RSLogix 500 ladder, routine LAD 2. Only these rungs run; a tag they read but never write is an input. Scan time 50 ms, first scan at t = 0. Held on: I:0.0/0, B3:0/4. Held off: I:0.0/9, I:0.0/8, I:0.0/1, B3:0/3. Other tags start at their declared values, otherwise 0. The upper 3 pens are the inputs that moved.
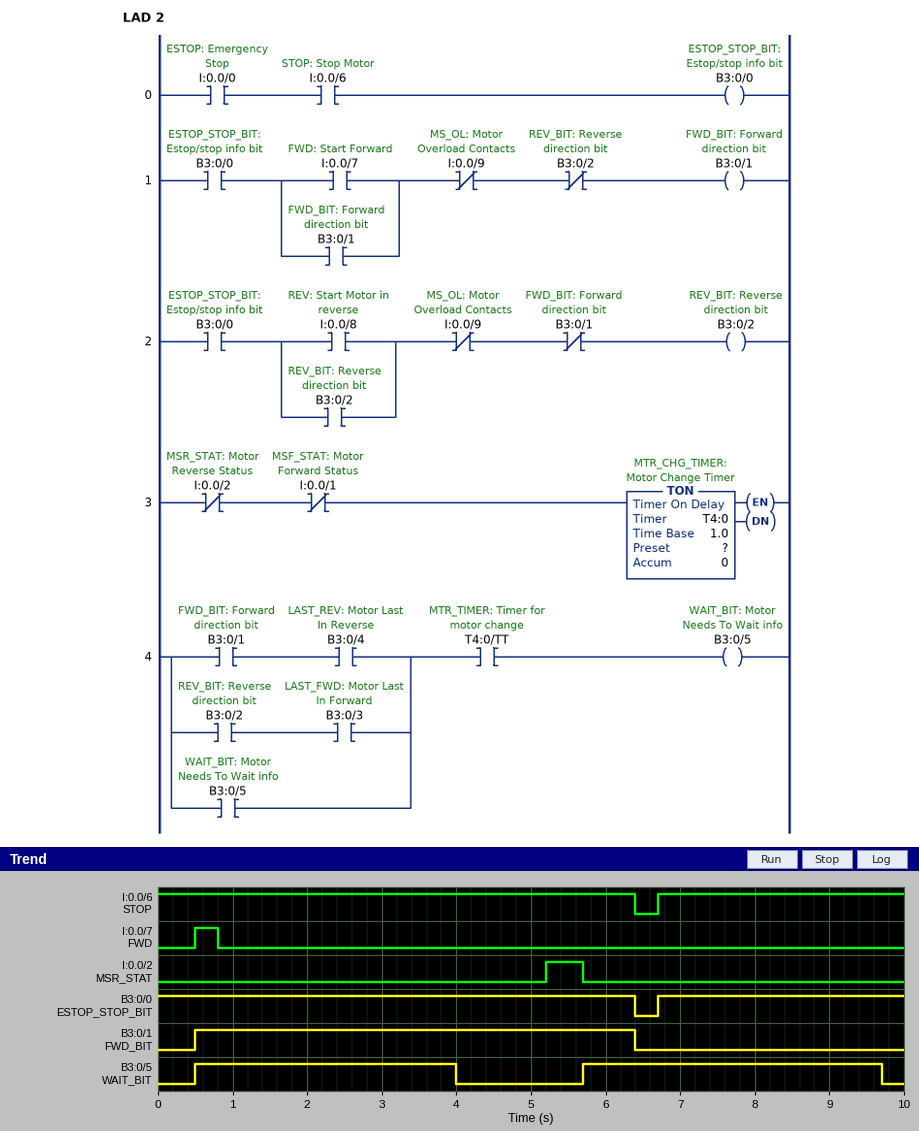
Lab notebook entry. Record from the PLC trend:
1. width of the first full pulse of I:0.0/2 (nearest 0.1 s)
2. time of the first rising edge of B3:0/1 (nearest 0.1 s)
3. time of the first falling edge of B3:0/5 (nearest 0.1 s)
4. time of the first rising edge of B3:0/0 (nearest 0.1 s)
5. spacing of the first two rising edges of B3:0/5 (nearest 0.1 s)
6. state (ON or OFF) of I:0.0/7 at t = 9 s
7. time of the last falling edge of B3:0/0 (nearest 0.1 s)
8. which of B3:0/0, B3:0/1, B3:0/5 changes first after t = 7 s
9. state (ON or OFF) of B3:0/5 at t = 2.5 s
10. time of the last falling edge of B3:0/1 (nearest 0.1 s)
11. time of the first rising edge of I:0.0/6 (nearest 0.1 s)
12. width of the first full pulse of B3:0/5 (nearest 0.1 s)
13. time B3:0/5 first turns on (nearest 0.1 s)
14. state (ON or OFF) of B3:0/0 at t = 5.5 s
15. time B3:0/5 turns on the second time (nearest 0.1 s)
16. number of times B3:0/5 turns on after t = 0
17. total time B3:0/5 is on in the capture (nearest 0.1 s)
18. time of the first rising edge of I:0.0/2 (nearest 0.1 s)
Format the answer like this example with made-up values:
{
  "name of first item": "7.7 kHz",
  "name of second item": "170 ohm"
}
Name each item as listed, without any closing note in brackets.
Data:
{
  "width of the first full pulse of I:0.0/2": "0.5 s",
  "time of the first rising edge of B3:0/1": "0.5 s",
  "time of the first falling edge of B3:0/5": "4.0 s",
  "time of the first rising edge of B3:0/0": "6.7 s",
  "spacing of the first two rising edges of B3:0/5": "5.2 s",
  "state (ON or OFF) of I:0.0/7 at t = 9 s": "OFF",
  "time of the last falling edge of B3:0/0": "6.4 s",
  "which of B3:0/0, B3:0/1, B3:0/5 changes first after t = 7 s": "B3:0/5",
  "state (ON or OFF) of B3:0/5 at t = 2.5 s": "ON",
  "time of the last falling edge of B3:0/1": "6.4 s",
  "time of the first rising edge of I:0.0/6": "6.7 s",
  "width of the first full pulse of B3:0/5": "3.5 s",
  "time B3:0/5 first turns on": "0.5 s",
  "state (ON or OFF) of B3:0/0 at t = 5.5 s": "ON",
  "time B3:0/5 turns on the second time": "5.7 s",
  "number of times B3:0/5 turns on after t = 0": "2",
  "total time B3:0/5 is on in the capture": "7.5 s",
  "time of the first rising edge of I:0.0/2": "5.2 s"
}
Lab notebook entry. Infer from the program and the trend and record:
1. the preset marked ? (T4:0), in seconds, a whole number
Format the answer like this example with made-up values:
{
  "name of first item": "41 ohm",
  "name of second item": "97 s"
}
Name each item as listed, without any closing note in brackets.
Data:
{
  "the preset marked ? (T4:0), in seconds, a whole number": "4 s"
}
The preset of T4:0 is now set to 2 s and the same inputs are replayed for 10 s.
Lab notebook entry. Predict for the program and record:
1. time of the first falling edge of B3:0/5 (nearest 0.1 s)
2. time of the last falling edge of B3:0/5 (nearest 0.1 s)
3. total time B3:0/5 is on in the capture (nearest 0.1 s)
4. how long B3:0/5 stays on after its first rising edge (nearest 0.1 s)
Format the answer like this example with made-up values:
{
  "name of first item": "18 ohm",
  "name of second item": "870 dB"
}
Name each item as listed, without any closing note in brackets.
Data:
{
  "time of the first falling edge of B3:0/5": "2.0 s",
  "time of the last falling edge of B3:0/5": "7.7 s",
  "total time B3:0/5 is on in the capture": "3.5 s",
  "how long B3:0/5 stays on after its first rising edge": "1.5 s"
}
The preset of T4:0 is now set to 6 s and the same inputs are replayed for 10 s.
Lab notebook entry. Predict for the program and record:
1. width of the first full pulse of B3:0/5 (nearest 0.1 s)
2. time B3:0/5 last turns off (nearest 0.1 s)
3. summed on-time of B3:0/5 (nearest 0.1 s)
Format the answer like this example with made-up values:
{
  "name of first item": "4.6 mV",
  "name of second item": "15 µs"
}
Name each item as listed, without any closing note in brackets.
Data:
{
  "width of the first full pulse of B3:0/5": "4.7 s",
  "time B3:0/5 last turns off": "5.2 s",
  "summed on-time of B3:0/5": "9.0 s"
}
